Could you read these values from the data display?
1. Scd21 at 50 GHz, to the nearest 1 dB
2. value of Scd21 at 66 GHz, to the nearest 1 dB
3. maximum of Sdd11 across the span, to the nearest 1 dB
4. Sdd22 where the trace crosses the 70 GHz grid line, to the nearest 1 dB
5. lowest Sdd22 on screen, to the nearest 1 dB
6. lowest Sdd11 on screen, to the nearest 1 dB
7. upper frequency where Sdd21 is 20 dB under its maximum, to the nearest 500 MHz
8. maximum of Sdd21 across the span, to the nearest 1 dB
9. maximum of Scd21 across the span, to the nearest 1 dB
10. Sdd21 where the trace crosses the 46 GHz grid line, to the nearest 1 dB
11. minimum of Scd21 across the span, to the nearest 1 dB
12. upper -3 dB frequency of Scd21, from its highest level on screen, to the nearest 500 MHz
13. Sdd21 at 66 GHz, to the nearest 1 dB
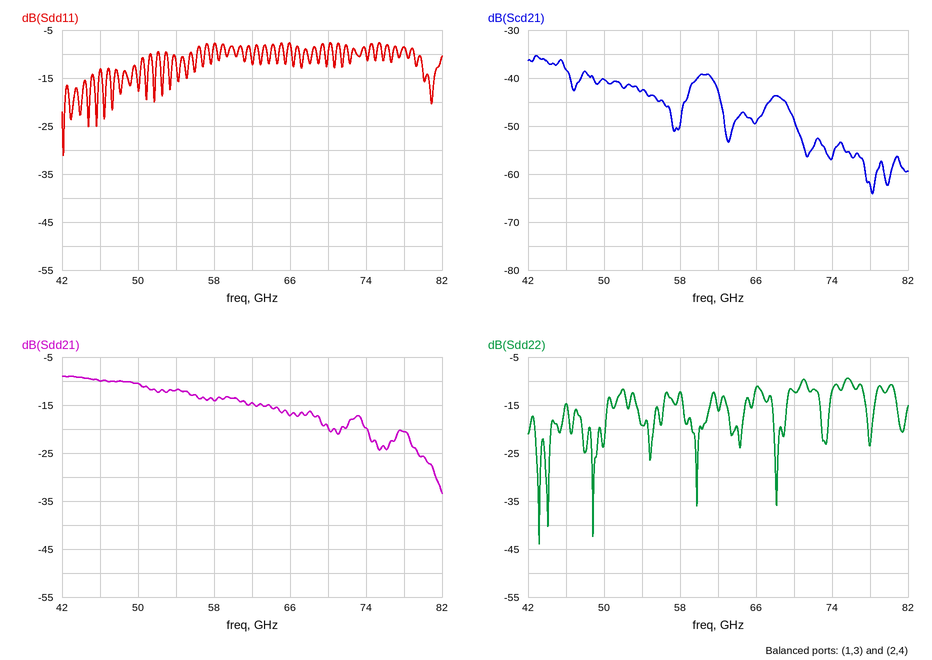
-40 dB
-49 dB
-8 dB
-12 dB
-44 dB
-31 dB
81.0 GHz
-9 dB
-35 dB
-10 dB
-64 dB
46.0 GHz
-17 dB
